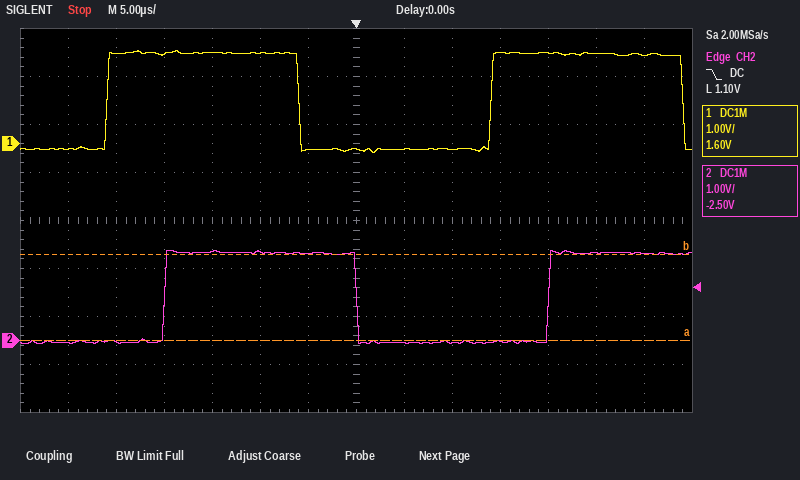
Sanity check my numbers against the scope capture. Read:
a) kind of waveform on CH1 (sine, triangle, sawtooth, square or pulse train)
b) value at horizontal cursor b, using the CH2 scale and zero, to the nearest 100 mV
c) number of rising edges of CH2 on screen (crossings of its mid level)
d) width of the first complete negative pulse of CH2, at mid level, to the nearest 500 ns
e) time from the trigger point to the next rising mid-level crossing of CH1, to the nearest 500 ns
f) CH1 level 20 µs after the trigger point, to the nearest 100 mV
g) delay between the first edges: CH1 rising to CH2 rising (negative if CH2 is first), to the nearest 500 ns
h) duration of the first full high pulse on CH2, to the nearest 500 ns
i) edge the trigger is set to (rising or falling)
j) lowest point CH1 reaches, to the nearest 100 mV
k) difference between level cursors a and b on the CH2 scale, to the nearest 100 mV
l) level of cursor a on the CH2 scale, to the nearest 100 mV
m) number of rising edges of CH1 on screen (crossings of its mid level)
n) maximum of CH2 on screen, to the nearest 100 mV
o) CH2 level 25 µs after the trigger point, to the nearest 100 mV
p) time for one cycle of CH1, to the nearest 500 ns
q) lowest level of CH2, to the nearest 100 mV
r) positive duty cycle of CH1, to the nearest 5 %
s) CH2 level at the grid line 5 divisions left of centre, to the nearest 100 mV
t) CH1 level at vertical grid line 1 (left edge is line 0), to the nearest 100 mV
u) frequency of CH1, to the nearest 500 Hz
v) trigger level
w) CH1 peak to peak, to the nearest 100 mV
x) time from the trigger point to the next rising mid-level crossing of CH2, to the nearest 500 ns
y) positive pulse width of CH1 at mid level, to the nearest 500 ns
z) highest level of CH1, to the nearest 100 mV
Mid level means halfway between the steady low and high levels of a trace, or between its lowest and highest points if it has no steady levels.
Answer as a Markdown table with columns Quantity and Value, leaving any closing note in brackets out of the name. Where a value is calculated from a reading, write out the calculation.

| Quantity | Value |
|---|---|
| kind of waveform on CH1 | square |
| value at horizontal cursor b, using the CH2 scale and zero, to the nearest 100 mV | 1.8 V |
| number of rising edges of CH2 on screen | 2 |
| width of the first complete negative pulse of CH2, at mid level, to the nearest 500 ns | 20.0 µs |
| time from the trigger point to the next rising mid-level crossing of CH1, to the nearest 500 ns | 14.0 µs |
| CH1 level 20 µs after the trigger point, to the nearest 100 mV | 1.9 V |
| delay between the first edges: CH1 rising to CH2 rising (negative if CH2 is first), to the nearest 500 ns | +6.0 µs |
| duration of the first full high pulse on CH2, to the nearest 500 ns | 20.0 µs |
| edge the trigger is set to | falling |
| lowest point CH1 reaches, to the nearest 100 mV | -200 mV |
| difference between level cursors a and b on the CH2 scale, to the nearest 100 mV | 1.8 V |
| level of cursor a on the CH2 scale, to the nearest 100 mV | 0.0 V |
| number of rising edges of CH1 on screen | 2 |
| maximum of CH2 on screen, to the nearest 100 mV | 1.9 V |
| CH2 level 25 µs after the trigger point, to the nearest 100 mV | 1.8 V |
| time for one cycle of CH1, to the nearest 500 ns | 40.0 µs |
| lowest level of CH2, to the nearest 100 mV | -100 mV |
| positive duty cycle of CH1, to the nearest 5 % | 20.0 µs / 40.0 µs ≈ 50 % |
| CH2 level at the grid line 5 divisions left of centre, to the nearest 100 mV | 0.0 V |
| CH1 level at vertical grid line 1 (left edge is line 0), to the nearest 100 mV | -100 mV |
| frequency of CH1, to the nearest 500 Hz | 1 / 40.0 µs ≈ 25.0 kHz |
| trigger level | 1.10 V |
| CH1 peak to peak, to the nearest 100 mV | 1.9 V − (-200 mV) = 2.1 V |
| time from the trigger point to the next rising mid-level crossing of CH2, to the nearest 500 ns | 20.0 µs |
| positive pulse width of CH1 at mid level, to the nearest 500 ns | 20.0 µs |
| highest level of CH1, to the nearest 100 mV | 1.9 V |
